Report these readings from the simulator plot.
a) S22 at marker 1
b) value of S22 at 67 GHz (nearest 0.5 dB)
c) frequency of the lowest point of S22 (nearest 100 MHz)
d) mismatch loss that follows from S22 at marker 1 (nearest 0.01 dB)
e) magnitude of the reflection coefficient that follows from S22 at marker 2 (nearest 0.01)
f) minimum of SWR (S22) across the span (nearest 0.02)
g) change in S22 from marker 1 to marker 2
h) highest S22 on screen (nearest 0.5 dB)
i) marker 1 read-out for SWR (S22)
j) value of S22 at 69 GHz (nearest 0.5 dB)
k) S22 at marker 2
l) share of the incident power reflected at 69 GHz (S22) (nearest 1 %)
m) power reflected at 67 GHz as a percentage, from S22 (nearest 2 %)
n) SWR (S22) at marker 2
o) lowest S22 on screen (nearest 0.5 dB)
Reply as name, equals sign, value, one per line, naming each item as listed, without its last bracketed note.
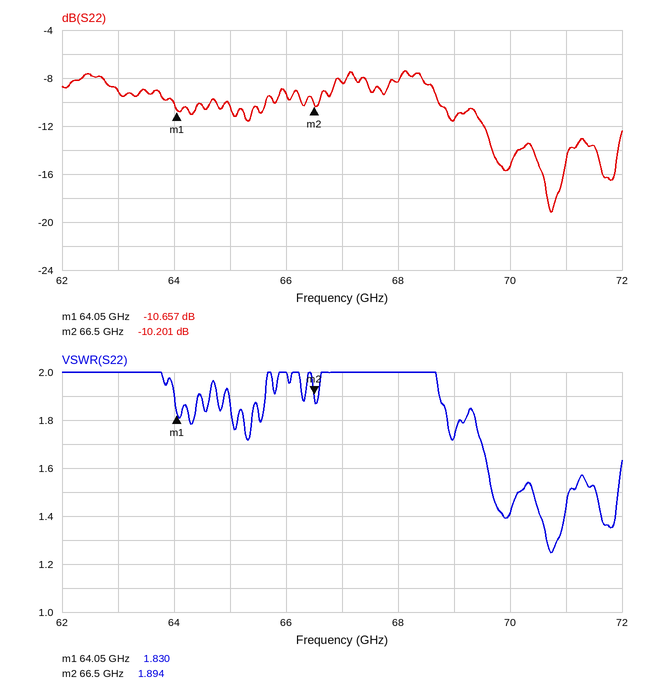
S22 at marker 1 = -10.657 dB
value of S22 at 67 GHz = -8.5 dB
frequency of the lowest point of S22 = 70.7 GHz
mismatch loss that follows from S22 at marker 1 = 0.39 dB
magnitude of the reflection coefficient that follows from S22 at marker 2 = 0.31
minimum of SWR (S22) across the span = 1.24
change in S22 from marker 1 to marker 2 = 0.456 dB
highest S22 on screen = -7.5 dB
marker 1 read-out for SWR = 1.830
value of S22 at 69 GHz = -11.5 dB
S22 at marker 2 = -10.201 dB
share of the incident power reflected at 69 GHz (S22) = 7 %
power reflected at 67 GHz as a percentage, from S22 = 14 %
SWR (S22) at marker 2 = 1.894
lowest S22 on screen = -19.0 dB
